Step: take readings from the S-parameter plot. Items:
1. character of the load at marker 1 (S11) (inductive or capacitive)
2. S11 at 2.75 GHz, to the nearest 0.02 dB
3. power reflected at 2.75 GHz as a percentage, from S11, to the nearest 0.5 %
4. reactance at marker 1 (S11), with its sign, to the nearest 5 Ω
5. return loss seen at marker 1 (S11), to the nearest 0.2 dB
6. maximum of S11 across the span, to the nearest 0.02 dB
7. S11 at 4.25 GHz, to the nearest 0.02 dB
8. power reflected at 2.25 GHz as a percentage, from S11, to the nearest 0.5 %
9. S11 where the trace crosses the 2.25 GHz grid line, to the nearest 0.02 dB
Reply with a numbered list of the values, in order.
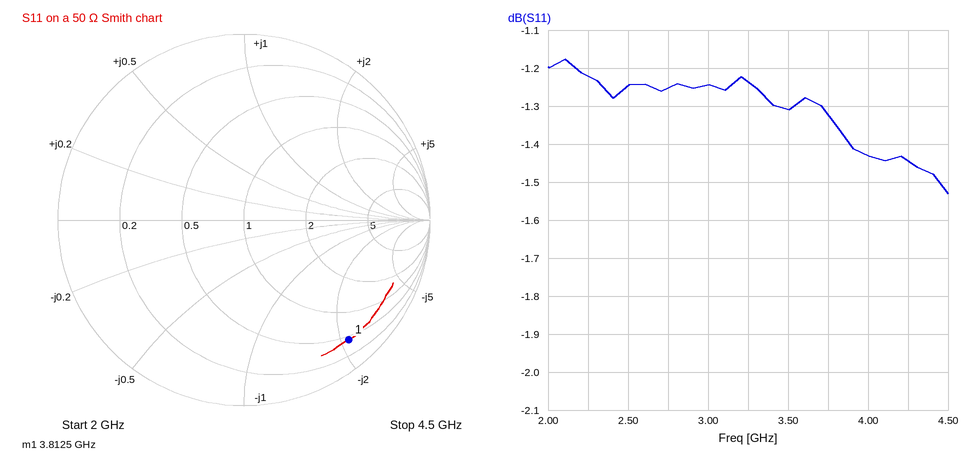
1. capacitive
2. -1.26 dB
3. 75.0 %
4. -105 Ω
5. 1.4 dB
6. -1.18 dB
7. -1.44 dB
8. 75.5 %
9. -1.22 dB
